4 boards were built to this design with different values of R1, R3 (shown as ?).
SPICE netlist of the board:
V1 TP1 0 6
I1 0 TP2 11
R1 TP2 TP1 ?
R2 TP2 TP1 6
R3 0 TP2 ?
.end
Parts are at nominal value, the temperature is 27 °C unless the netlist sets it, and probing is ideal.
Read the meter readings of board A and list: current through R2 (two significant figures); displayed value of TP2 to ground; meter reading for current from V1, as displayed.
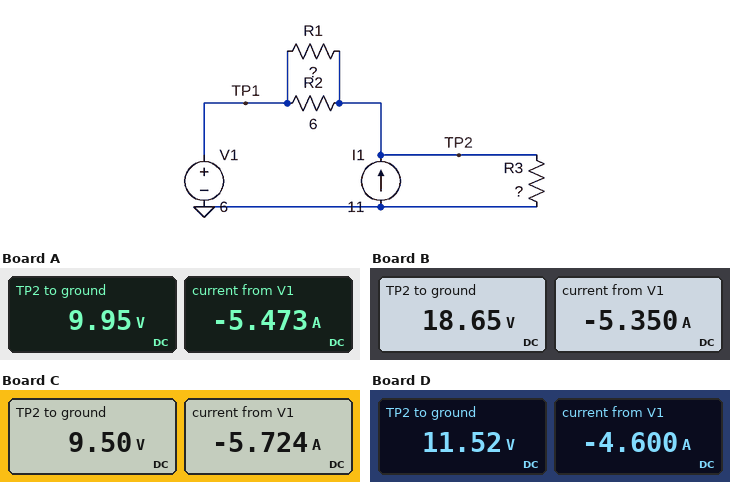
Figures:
660 mA
9.95 V
-5.473 A
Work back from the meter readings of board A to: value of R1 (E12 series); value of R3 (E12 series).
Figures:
0.82 Ω
1.8 Ω
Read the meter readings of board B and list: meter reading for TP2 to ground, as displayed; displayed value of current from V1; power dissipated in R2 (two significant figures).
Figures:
18.65 V
-5.350 A
27 W
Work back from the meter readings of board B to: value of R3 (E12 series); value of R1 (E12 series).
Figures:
3.3 Ω
3.9 Ω
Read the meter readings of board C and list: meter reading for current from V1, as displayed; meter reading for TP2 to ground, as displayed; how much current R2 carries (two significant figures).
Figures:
-5.724 A
9.50 V
580 mA
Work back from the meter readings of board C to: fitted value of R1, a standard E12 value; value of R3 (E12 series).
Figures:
0.68 Ω
1.8 Ω
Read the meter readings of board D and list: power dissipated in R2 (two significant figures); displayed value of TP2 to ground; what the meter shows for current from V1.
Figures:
5.1 W
11.52 V
-4.600 A
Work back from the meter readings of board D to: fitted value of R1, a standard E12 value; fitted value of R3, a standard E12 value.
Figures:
1.5 Ω
1.8 Ω
